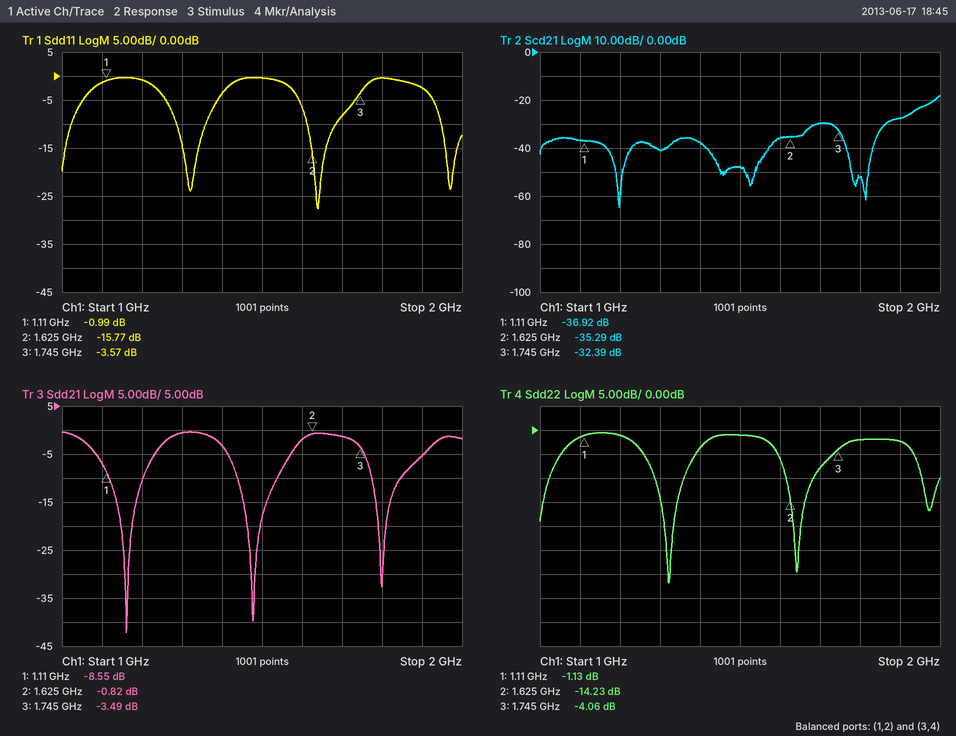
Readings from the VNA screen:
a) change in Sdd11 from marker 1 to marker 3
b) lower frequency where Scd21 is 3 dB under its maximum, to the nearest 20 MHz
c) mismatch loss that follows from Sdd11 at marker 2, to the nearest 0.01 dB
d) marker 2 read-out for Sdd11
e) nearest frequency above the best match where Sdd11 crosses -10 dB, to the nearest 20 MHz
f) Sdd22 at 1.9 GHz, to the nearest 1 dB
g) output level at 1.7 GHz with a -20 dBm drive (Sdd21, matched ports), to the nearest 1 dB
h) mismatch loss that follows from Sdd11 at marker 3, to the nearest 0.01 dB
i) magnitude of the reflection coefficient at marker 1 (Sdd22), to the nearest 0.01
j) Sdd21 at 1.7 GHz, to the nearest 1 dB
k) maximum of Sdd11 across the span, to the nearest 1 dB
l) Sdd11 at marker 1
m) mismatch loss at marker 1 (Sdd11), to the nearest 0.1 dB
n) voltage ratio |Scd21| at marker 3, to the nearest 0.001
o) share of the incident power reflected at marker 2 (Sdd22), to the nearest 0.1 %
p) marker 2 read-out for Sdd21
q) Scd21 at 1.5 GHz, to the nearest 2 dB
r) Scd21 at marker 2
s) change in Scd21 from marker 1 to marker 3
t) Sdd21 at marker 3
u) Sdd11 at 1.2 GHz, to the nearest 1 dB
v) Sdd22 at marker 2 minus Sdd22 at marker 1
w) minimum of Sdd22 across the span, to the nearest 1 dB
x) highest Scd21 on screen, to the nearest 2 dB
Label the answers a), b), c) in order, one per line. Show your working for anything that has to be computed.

a) -3.57 − (-0.99) = -2.58 dB
b) 1.98 GHz
c) −10 log10(1 − 10^(-15.77/10)) ≈ 0.12 dB
d) -15.77 dB
e) 1.68 GHz
f) -2 dB
g) -20 dBm + (-1 dB) = -21 dBm
h) −10 log10(1 − 10^(-3.57/10)) ≈ 2.51 dB
i) 10^(-1.13/20) ≈ 0.88
j) -1 dB
k) 0 dB
l) -0.99 dB
m) −10 log10(1 − 10^(-0.99/10)) ≈ 6.9 dB
n) 10^(-32.39/20) ≈ 0.024
o) 10^(-14.23/10) ≈ 3.8 %
p) -0.82 dB
q) -48 dB
r) -35.29 dB
s) -32.39 − (-36.92) = 4.53 dB
t) -3.49 dB
u) -1 dB
v) -14.23 − (-1.13) = -13.10 dB
w) -32 dB
x) -18 dB
